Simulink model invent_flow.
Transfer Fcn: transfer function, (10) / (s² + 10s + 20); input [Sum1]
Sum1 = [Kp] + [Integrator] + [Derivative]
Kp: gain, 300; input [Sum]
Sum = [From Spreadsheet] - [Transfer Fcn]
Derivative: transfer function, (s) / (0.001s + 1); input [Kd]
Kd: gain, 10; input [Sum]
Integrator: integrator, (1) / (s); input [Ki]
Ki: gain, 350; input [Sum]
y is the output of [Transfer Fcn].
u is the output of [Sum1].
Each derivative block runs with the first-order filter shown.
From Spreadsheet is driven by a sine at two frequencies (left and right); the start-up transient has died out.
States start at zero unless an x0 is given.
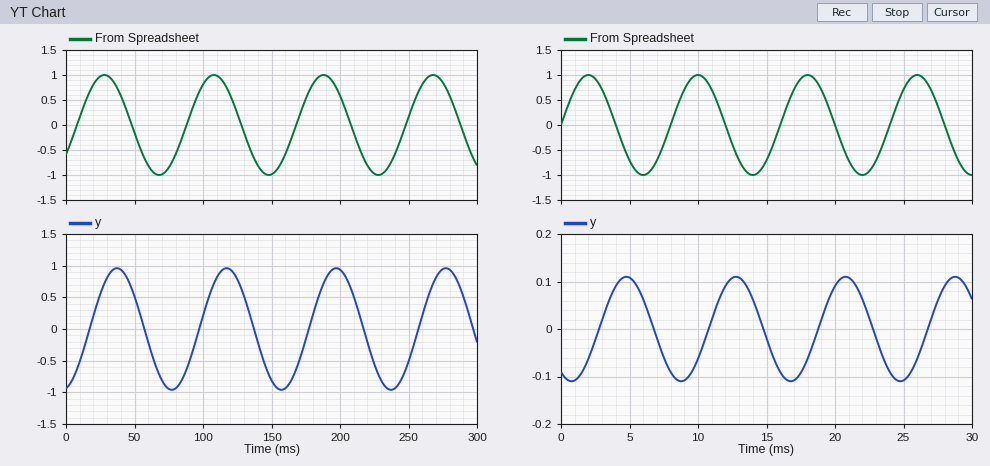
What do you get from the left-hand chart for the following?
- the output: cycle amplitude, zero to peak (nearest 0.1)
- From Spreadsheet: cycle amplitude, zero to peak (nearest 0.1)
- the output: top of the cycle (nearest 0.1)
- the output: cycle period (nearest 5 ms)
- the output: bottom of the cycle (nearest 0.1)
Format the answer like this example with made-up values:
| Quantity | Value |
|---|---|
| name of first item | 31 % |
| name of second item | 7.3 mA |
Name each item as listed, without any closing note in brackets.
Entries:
| Quantity | Value |
|---|---|
| the output: cycle amplitude, zero to peak | 1.0 |
| From Spreadsheet: cycle amplitude, zero to peak | 1.0 |
| the output: top of the cycle | 1.0 |
| the output: cycle period | 80 ms |
| the output: bottom of the cycle | -1.0 |
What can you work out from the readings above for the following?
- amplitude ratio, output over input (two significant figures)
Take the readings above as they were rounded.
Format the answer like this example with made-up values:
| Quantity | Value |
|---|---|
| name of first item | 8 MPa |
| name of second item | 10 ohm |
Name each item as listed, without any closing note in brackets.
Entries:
| Quantity | Value |
|---|---|
| amplitude ratio, output over input | 1.0 |
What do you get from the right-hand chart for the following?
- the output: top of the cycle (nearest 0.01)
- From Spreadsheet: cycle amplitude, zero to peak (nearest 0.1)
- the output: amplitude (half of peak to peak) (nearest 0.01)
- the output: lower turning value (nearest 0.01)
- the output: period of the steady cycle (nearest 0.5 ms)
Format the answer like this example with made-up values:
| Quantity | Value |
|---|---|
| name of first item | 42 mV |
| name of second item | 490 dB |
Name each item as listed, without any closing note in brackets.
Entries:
| Quantity | Value |
|---|---|
| the output: top of the cycle | 0.11 |
| From Spreadsheet: cycle amplitude, zero to peak | 1.0 |
| the output: amplitude (half of peak to peak) | 0.11 |
| the output: lower turning value | -0.11 |
| the output: period of the steady cycle | 8.0 ms |
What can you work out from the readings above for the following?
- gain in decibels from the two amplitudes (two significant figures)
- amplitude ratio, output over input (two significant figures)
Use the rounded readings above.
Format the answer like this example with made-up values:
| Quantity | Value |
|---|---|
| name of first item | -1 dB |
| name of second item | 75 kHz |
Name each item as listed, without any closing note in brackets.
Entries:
| Quantity | Value |
|---|---|
| gain in decibels from the two amplitudes | -19 dB |
| amplitude ratio, output over input | 0.11 |
